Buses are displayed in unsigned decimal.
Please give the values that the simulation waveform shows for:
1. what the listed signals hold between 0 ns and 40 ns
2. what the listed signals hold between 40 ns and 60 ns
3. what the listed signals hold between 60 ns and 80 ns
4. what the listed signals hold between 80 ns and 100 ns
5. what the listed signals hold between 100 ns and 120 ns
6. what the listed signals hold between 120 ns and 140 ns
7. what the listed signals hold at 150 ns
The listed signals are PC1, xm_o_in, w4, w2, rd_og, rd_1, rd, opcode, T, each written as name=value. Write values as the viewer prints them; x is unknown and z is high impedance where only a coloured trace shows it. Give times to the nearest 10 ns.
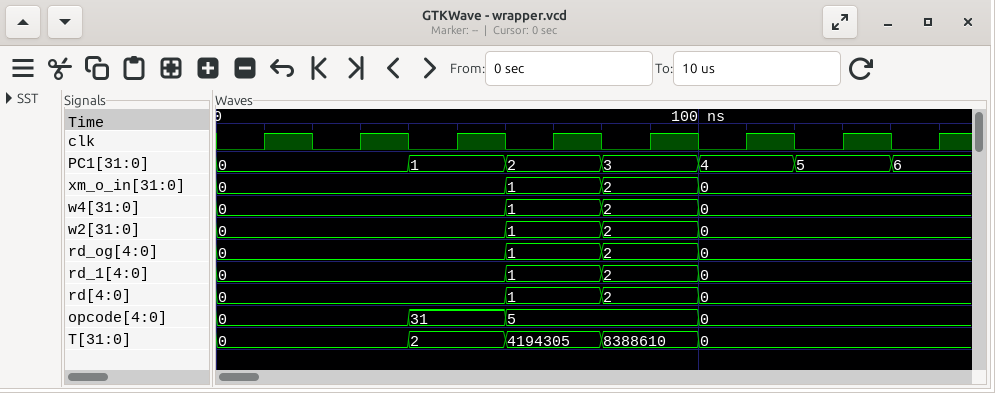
PC1=0, xm_o_in=0, w4=0, w2=0, rd_og=0, rd_1=0, rd=0, opcode=0, T=0
PC1=1, xm_o_in=0, w4=0, w2=0, rd_og=0, rd_1=0, rd=0, opcode=31, T=2
PC1=2, xm_o_in=1, w4=1, w2=1, rd_og=1, rd_1=1, rd=1, opcode=5, T=4194305
PC1=3, xm_o_in=2, w4=2, w2=2, rd_og=2, rd_1=2, rd=2, opcode=5, T=8388610
PC1=4, xm_o_in=0, w4=0, w2=0, rd_og=0, rd_1=0, rd=0, opcode=0, T=0
PC1=5, xm_o_in=0, w4=0, w2=0, rd_og=0, rd_1=0, rd=0, opcode=0, T=0
PC1=6, xm_o_in=0, w4=0, w2=0, rd_og=0, rd_1=0, rd=0, opcode=0, T=0
